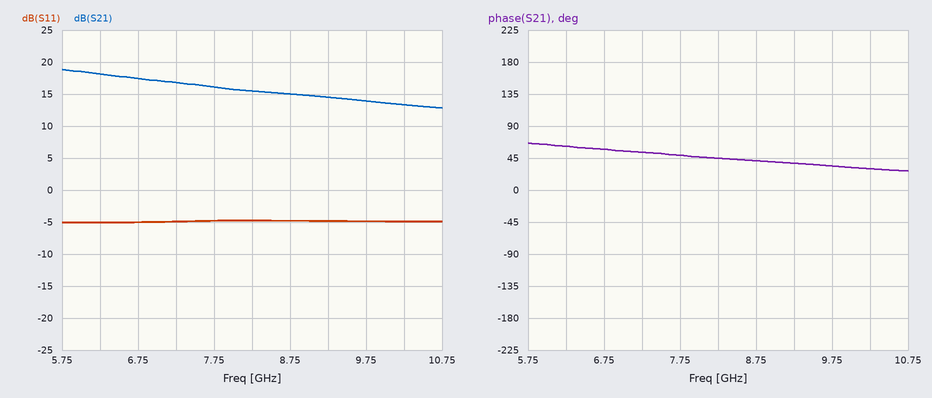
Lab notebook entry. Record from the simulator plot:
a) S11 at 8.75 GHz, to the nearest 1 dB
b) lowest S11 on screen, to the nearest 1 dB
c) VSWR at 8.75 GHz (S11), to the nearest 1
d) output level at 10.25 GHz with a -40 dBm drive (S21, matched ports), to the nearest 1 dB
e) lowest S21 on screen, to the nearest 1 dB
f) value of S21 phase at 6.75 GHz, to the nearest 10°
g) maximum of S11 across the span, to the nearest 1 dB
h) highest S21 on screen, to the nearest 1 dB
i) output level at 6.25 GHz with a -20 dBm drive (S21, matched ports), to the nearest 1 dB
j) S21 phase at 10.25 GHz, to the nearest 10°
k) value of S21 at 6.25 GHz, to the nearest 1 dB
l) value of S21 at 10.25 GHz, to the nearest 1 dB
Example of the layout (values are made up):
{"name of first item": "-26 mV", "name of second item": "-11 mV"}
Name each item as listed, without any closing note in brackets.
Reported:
{"S11 at 8.75 GHz, to the nearest 1 dB": "-5 dB", "lowest S11 on screen, to the nearest 1 dB": "-5 dB", "VSWR at 8.75 GHz (S11), to the nearest 1": "4", "output level at 10.25 GHz with a -40 dBm drive (S21, matched ports), to the nearest 1 dB": "-27 dBm", "lowest S21 on screen, to the nearest 1 dB": "13 dB", "value of S21 phase at 6.75 GHz, to the nearest 10°": "60°", "maximum of S11 across the span, to the nearest 1 dB": "-5 dB", "highest S21 on screen, to the nearest 1 dB": "19 dB", "output level at 6.25 GHz with a -20 dBm drive (S21, matched ports), to the nearest 1 dB": "-2 dBm", "S21 phase at 10.25 GHz, to the nearest 10°": "30°", "value of S21 at 6.25 GHz, to the nearest 1 dB": "18 dB", "value of S21 at 10.25 GHz, to the nearest 1 dB": "13 dB"}
